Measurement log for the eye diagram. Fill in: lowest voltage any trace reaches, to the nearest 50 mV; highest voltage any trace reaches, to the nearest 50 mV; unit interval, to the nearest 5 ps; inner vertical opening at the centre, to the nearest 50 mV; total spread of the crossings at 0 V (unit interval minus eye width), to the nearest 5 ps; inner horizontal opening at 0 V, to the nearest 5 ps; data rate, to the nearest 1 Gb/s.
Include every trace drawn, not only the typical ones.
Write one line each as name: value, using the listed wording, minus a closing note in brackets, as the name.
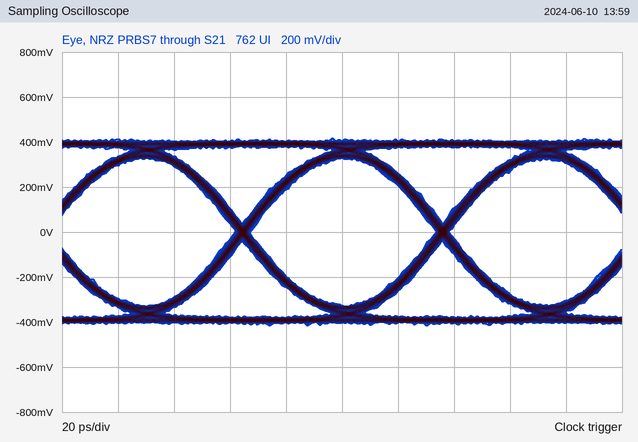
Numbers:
lowest voltage any trace reaches, to the nearest 50 mV: -400 mV
highest voltage any trace reaches, to the nearest 50 mV: 400 mV
unit interval, to the nearest 5 ps: 70 ps
inner vertical opening at the centre, to the nearest 50 mV: 650 mV
total spread of the crossings at 0 V (unit interval minus eye width), to the nearest 5 ps: 5 ps
inner horizontal opening at 0 V, to the nearest 5 ps: 65 ps
data rate, to the nearest 1 Gb/s: 14 Gb/s
